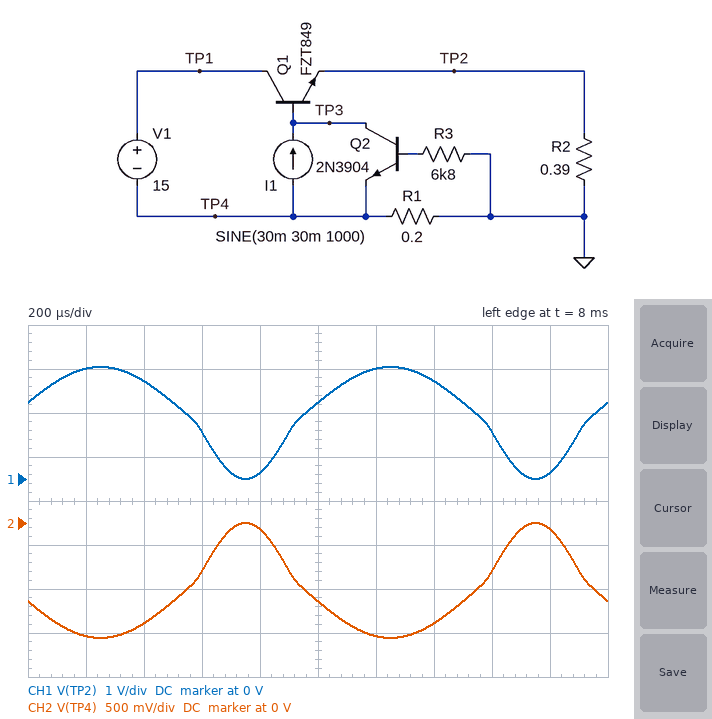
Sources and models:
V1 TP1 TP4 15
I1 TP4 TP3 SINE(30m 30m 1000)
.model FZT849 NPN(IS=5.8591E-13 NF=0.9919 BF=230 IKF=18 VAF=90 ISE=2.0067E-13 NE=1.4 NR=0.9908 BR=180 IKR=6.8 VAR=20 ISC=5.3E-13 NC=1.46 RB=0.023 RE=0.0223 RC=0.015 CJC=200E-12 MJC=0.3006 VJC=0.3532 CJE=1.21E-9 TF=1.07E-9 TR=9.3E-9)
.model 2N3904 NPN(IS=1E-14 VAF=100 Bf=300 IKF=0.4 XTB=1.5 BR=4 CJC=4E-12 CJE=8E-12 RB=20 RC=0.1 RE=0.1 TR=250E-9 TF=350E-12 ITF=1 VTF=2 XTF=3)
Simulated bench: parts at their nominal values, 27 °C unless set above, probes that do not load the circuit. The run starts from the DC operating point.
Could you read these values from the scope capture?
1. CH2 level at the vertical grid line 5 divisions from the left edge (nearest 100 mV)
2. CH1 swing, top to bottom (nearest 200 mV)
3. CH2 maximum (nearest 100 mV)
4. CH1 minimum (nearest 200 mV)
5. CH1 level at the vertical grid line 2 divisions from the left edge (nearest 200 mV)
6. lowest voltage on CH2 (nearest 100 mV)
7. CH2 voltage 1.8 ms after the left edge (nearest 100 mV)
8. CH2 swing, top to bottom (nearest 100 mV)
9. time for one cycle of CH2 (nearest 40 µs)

-900 mV
2.6 V
0 V
0 V
2.2 V
-1.3 V
-100 mV
1.3 V
1.00 ms
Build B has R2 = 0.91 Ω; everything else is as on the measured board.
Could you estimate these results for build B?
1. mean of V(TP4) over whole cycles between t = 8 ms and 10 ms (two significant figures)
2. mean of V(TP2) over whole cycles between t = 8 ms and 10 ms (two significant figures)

-770 mV
3.5 V
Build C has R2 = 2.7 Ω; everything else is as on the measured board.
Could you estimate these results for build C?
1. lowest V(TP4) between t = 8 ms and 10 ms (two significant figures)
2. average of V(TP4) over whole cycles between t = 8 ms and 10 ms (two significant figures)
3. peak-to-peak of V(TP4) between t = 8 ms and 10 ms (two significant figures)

-1.0 V
-690 mV
1.0 V
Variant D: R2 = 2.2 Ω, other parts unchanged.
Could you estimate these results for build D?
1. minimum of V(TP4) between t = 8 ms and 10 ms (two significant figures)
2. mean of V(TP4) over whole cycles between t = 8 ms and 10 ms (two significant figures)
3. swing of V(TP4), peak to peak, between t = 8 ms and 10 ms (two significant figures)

-1.2 V
-740 mV
1.2 V
